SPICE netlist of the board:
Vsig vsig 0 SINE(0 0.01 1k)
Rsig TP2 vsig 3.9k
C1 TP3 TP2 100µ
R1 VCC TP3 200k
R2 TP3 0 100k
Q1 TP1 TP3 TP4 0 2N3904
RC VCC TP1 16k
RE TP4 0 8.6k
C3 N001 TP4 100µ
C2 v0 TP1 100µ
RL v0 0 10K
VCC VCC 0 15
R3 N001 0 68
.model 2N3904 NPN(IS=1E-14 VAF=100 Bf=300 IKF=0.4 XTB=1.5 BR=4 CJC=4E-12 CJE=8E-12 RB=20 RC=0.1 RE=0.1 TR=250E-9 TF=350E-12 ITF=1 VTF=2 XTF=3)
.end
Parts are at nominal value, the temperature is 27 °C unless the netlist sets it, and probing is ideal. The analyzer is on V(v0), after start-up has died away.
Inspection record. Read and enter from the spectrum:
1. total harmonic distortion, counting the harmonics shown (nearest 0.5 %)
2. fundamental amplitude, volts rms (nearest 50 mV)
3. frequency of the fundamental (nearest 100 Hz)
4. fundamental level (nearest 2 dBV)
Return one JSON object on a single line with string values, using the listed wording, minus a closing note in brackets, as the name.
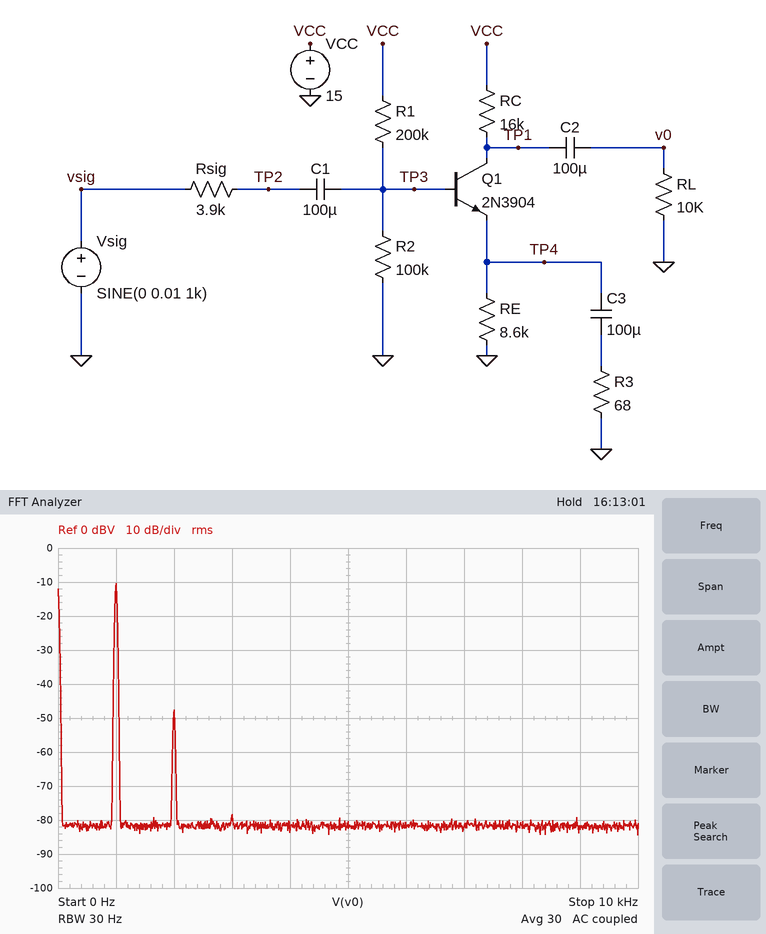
{"total harmonic distortion, counting the harmonics shown": "1.5 %", "fundamental amplitude, volts rms": "300 mV", "frequency of the fundamental": "1.0 kHz", "fundamental level": "-10 dBV"}
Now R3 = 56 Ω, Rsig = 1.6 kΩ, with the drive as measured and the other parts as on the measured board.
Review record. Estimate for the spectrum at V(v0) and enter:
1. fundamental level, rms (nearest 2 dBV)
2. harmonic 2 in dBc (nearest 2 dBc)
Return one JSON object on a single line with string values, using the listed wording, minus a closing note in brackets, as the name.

{"fundamental level, rms": "-8 dBV", "harmonic 2 in dBc": "-34 dBc"}
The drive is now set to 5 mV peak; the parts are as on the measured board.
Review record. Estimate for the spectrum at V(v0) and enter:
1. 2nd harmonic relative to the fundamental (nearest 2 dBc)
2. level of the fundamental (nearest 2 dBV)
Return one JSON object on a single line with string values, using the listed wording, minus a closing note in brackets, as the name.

{"2nd harmonic relative to the fundamental": "-44 dBc", "level of the fundamental": "-16 dBV"}
